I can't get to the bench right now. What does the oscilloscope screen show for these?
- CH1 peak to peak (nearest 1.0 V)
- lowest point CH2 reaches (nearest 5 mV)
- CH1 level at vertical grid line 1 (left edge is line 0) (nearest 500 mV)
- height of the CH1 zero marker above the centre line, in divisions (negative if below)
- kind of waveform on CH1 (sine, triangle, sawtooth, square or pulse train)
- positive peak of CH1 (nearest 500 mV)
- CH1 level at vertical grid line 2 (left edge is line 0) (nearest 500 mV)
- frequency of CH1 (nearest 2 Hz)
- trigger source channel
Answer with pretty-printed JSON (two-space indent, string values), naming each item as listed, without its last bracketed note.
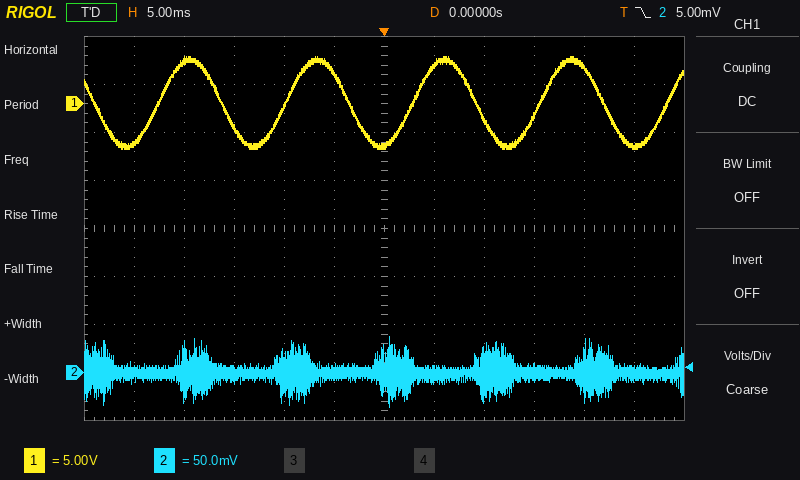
{
  "CH1 peak to peak": "10.0 V",
  "lowest point CH2 reaches": "-35 mV",
  "CH1 level at vertical grid line 1 (left edge is line 0)": "-4.0 V",
  "height of the CH1 zero marker above the centre line, in divisions": "+2.6 div",
  "kind of waveform on CH1": "sine",
  "positive peak of CH1": "5.0 V",
  "CH1 level at vertical grid line 2 (left edge is line 0)": "4.5 V",
  "frequency of CH1": "78 Hz",
  "trigger source channel": "CH2"
}
